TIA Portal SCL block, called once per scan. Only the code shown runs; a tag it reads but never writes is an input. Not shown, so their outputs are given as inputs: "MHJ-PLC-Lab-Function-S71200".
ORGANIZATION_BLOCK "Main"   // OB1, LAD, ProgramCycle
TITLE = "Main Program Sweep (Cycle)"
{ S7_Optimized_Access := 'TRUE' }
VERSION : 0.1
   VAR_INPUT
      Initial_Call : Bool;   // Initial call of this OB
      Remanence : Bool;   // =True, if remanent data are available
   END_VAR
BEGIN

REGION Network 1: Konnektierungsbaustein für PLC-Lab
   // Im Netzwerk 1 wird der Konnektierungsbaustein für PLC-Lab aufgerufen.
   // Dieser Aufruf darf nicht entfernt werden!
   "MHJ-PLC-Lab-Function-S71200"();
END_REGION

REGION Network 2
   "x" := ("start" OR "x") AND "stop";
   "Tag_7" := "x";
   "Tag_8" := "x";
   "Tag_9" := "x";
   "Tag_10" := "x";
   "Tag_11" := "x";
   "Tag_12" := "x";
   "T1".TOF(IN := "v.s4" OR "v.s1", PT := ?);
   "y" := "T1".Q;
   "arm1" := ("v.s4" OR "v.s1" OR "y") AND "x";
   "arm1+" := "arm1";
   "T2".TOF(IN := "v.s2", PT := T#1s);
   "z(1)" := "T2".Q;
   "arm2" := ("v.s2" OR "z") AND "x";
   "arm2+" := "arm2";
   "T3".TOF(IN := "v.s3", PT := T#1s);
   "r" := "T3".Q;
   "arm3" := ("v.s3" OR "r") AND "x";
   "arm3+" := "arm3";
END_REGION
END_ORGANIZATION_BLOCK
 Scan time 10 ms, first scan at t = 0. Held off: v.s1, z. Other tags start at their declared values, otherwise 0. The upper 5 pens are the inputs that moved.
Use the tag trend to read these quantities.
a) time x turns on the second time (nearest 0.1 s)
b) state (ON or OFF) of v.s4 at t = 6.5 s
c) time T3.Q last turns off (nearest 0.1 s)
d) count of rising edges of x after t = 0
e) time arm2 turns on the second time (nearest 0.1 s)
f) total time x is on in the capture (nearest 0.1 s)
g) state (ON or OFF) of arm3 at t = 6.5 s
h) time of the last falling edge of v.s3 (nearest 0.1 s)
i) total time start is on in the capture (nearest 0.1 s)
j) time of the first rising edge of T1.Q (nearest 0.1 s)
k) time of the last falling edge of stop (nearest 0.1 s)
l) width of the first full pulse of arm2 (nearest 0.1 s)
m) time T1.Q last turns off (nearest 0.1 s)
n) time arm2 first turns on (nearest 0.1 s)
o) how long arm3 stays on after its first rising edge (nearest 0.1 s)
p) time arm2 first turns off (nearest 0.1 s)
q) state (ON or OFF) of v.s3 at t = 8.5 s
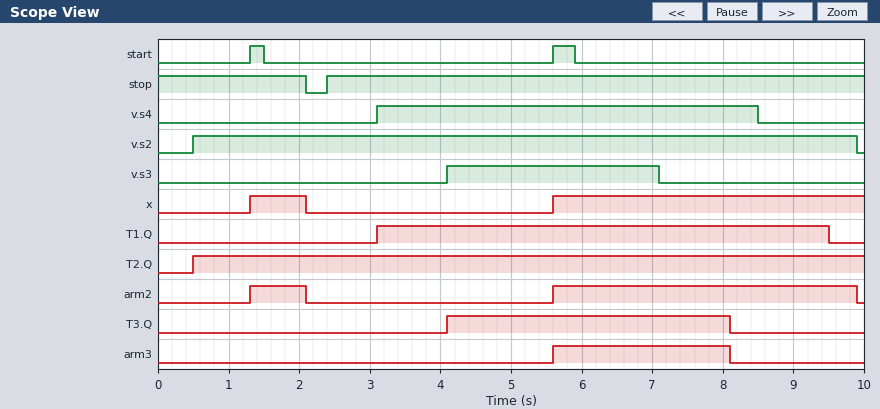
5.6 s
ON
8.1 s
2
5.6 s
5.2 s
ON
7.1 s
0.5 s
3.1 s
2.1 s
0.8 s
9.5 s
1.3 s
2.5 s
2.1 s
OFF
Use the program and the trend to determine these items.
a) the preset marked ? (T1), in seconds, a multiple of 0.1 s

1.0 s
